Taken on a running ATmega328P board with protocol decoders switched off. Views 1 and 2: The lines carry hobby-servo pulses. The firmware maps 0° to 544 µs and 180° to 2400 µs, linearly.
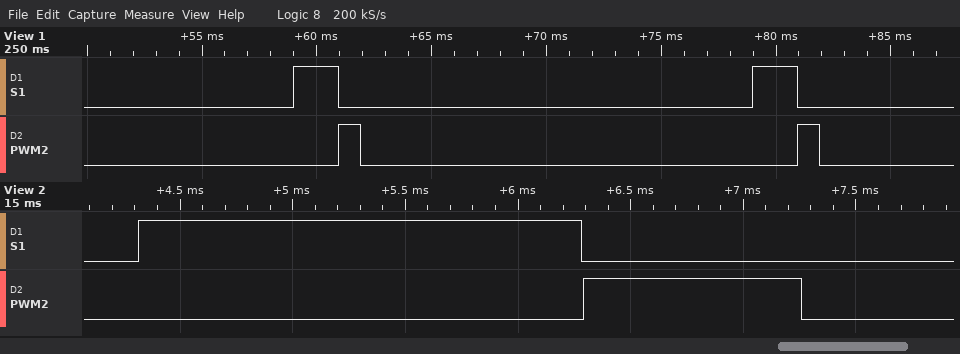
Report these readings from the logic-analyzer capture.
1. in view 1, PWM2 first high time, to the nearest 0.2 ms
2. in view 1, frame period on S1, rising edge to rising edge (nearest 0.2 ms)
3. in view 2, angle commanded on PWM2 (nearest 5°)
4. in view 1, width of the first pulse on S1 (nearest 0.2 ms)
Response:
1.0 ms
20.0 ms
40°
2.0 ms
